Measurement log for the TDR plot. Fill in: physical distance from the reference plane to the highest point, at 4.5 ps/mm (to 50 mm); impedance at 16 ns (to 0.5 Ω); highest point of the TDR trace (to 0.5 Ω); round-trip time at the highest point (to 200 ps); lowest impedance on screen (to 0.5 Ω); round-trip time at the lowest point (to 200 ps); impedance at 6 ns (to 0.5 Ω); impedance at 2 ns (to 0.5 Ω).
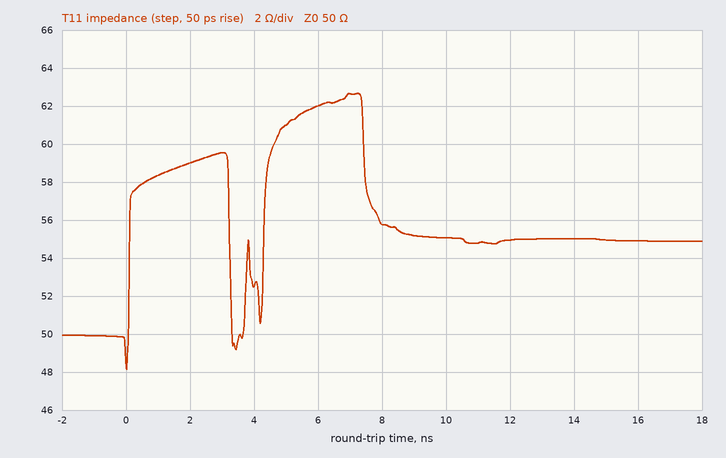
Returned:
800 mm
55.0 Ω
62.5 Ω
7.2 ns
48.0 Ω
0.0 ns
62.0 Ω
59.0 Ω
